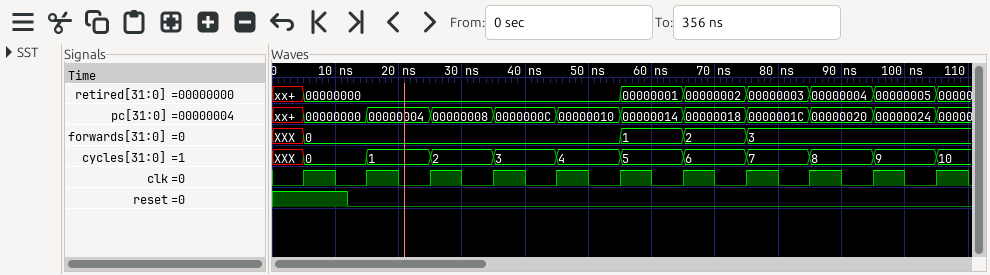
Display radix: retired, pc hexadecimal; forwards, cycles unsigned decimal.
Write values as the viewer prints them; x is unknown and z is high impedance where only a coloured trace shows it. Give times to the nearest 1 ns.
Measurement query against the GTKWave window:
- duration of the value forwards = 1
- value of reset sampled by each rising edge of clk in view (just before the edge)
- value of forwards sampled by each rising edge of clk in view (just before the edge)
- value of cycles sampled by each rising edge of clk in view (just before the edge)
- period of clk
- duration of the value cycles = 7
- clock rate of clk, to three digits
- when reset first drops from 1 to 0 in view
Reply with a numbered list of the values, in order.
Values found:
1. 10 ns
2. 1 0 0 0 0 0 0 0 0 0 0
3. XXX, 0, 0, 0, 0, 0, 1, 2, 3, 3, 3
4. XXX, 0, 1, 2, 3, 4, 5, 6, 7, 8, 9
5. 10 ns
6. 10 ns
7. 100 MHz
8. 12 ns
